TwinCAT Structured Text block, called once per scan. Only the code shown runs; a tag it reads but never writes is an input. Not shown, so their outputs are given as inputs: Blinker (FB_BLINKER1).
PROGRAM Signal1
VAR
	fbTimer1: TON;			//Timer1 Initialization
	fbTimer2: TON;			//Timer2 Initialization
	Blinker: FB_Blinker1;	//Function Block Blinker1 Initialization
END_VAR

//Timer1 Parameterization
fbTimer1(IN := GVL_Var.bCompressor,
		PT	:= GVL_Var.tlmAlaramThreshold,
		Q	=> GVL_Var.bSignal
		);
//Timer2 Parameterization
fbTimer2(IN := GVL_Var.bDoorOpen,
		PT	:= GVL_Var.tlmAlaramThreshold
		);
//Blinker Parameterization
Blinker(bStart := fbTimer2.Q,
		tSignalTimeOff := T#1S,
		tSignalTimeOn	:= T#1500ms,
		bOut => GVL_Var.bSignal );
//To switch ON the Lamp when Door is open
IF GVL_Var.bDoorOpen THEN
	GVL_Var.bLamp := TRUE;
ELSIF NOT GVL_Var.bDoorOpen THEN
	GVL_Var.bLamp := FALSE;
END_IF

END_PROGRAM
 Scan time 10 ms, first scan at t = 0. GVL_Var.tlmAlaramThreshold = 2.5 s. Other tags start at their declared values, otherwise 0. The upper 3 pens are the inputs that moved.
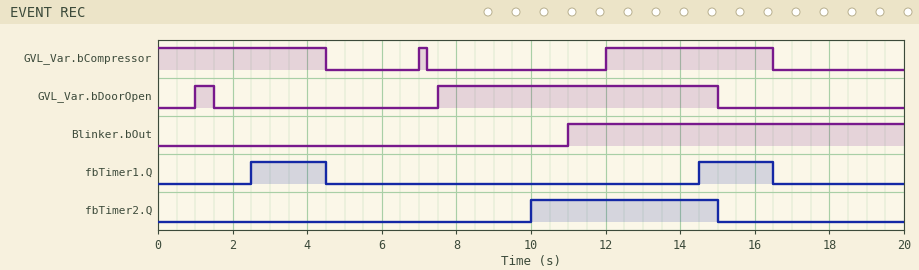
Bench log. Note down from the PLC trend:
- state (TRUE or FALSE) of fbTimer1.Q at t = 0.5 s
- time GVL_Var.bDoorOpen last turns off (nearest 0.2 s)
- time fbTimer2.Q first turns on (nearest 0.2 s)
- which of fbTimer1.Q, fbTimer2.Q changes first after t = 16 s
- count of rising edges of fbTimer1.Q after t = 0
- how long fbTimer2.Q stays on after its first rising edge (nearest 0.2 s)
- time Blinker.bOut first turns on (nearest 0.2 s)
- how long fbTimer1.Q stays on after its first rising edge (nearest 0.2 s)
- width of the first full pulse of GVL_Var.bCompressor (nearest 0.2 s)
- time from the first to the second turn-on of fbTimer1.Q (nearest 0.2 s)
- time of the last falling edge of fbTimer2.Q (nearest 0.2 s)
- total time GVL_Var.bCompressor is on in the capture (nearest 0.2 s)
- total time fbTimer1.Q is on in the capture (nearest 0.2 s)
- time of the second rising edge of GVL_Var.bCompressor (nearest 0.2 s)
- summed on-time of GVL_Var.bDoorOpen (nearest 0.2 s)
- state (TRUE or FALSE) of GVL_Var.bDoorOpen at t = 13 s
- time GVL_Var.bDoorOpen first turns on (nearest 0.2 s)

FALSE
15.0 s
10.0 s
fbTimer1.Q
2
5.0 s
11.0 s
2.0 s
0.2 s
12.0 s
15.0 s
9.2 s
4.0 s
12.0 s
8.0 s
TRUE
1.0 s
